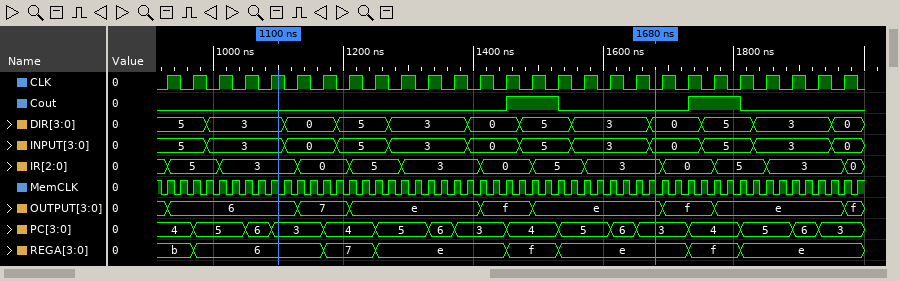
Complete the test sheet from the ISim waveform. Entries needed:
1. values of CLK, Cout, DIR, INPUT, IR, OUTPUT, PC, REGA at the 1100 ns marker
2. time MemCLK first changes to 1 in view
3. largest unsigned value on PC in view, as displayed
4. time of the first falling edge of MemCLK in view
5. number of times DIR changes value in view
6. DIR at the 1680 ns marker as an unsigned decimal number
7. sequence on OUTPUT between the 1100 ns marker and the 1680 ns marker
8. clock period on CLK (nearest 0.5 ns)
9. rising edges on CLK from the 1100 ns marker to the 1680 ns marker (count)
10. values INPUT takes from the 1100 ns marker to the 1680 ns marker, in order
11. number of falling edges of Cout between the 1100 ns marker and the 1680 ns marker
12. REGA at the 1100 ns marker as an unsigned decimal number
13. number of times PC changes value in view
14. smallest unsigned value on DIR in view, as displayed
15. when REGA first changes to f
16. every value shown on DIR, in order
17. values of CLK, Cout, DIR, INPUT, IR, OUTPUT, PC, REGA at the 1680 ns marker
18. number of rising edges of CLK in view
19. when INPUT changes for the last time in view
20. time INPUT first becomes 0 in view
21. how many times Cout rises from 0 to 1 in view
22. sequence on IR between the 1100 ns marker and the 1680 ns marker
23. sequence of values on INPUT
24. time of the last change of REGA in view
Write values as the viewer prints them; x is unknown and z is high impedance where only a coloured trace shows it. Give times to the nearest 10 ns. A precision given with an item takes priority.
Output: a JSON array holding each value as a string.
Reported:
["CLK=1, Cout=0, DIR=3, INPUT=3, IR=3, OUTPUT=6, PC=3, REGA=6", "930 ns", "6", "920 ns", "11", "0", "6, 7, e, f, e", "40 ns", "14", "3, 0, 5, 3, 0, 5, 3, 0", "1", "6", "15", "0", "1450 ns", "5, 3, 0, 5, 3, 0, 5, 3, 0, 5, 3, 0", "CLK=0, Cout=0, DIR=0, INPUT=0, IR=3, OUTPUT=e, PC=3, REGA=e", "27", "1950 ns", "1110 ns", "2", "3, 0, 5, 3, 0, 5, 3", "5, 3, 0, 5, 3, 0, 5, 3, 0, 5, 3, 0", "1810 ns"]
